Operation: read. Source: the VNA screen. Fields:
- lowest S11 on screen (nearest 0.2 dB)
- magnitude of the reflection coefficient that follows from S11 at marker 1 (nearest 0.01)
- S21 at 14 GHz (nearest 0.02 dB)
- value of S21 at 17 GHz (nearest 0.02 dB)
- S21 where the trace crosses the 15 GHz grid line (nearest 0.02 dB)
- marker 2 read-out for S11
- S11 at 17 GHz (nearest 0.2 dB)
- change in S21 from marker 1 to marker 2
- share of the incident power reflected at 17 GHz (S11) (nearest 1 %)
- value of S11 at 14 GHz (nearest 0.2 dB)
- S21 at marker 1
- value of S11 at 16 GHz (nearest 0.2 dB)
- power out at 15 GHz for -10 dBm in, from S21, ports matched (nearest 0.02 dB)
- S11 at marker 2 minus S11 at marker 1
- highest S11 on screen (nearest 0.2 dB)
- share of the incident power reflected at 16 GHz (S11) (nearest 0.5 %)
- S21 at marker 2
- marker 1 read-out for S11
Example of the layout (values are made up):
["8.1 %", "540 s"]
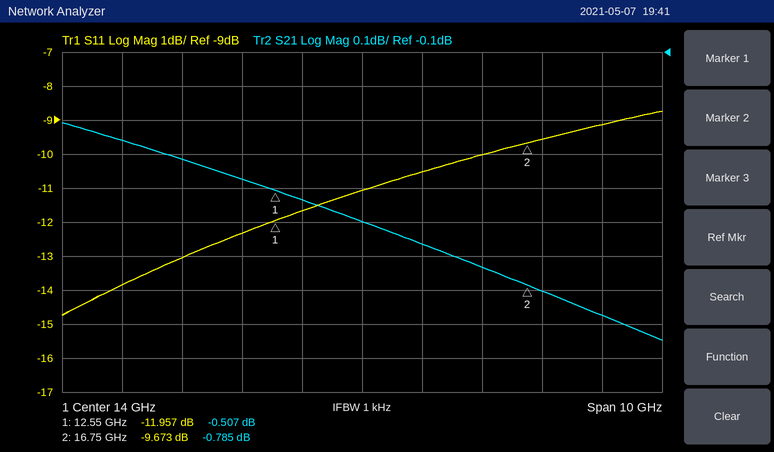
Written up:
["-14.8 dB", "0.25", "-0.60 dB", "-0.80 dB", "-0.66 dB", "-9.673 dB", "-9.6 dB", "-0.278 dB", "11 %", "-11.0 dB", "-0.507 dB", "-10.0 dB", "-10.66 dBm", "2.284 dB", "-8.8 dB", "10.0 %", "-0.785 dB", "-11.957 dB"]
